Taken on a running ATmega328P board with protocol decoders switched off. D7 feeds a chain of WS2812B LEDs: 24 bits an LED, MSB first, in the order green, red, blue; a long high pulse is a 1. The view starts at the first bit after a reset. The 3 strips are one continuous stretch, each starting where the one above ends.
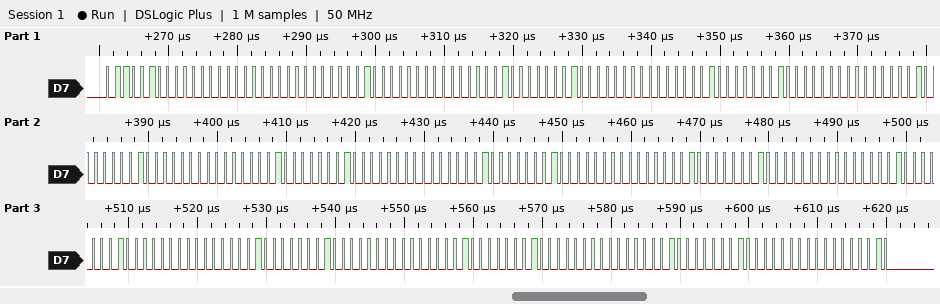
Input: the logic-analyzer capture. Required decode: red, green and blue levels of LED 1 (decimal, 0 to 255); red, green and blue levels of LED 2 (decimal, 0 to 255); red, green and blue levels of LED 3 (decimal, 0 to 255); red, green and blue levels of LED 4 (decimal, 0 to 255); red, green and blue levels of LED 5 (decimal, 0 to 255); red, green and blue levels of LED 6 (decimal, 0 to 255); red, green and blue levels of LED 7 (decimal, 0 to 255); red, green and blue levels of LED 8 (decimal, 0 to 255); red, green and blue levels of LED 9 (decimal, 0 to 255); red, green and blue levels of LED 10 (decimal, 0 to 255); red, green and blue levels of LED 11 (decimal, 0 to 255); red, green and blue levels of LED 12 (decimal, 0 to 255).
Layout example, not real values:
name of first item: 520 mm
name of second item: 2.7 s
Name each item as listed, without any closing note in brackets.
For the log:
red, green and blue levels of LED 1: 0, 100, 0
red, green and blue levels of LED 2: 0, 2, 2
red, green and blue levels of LED 3: 0, 2, 2
red, green and blue levels of LED 4: 0, 2, 2
red, green and blue levels of LED 5: 0, 2, 2
red, green and blue levels of LED 6: 0, 2, 2
red, green and blue levels of LED 7: 0, 2, 2
red, green and blue levels of LED 8: 0, 2, 2
red, green and blue levels of LED 9: 0, 2, 2
red, green and blue levels of LED 10: 0, 2, 2
red, green and blue levels of LED 11: 0, 2, 2
red, green and blue levels of LED 12: 0, 2, 2
